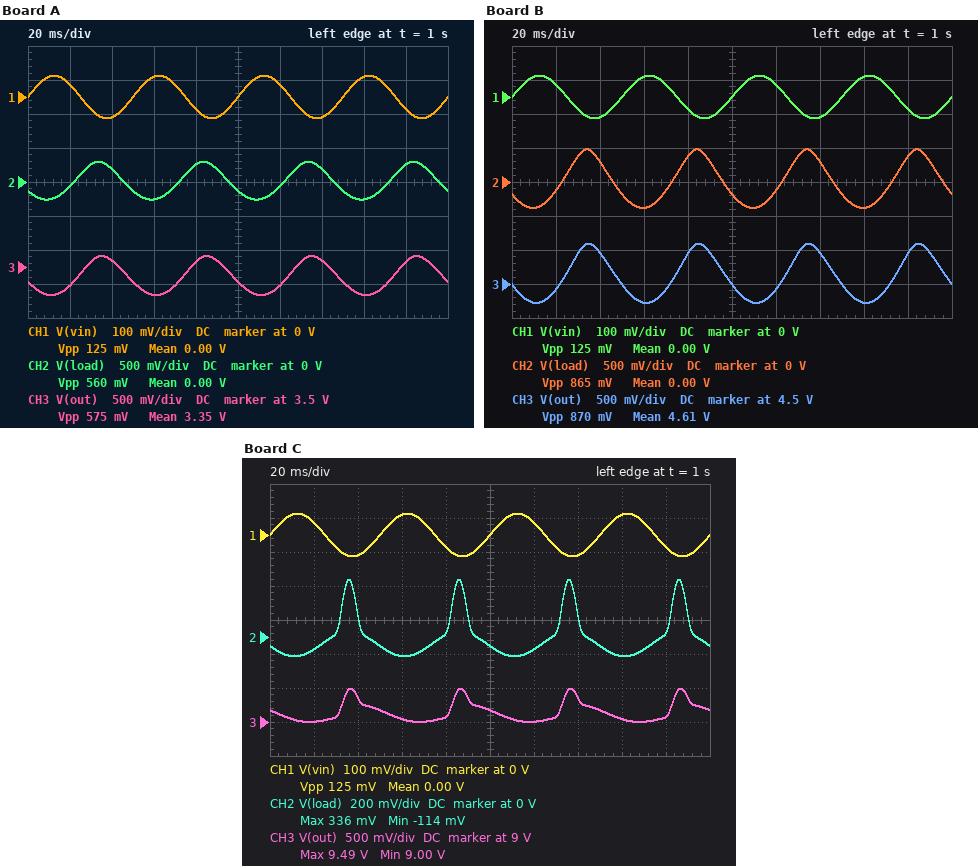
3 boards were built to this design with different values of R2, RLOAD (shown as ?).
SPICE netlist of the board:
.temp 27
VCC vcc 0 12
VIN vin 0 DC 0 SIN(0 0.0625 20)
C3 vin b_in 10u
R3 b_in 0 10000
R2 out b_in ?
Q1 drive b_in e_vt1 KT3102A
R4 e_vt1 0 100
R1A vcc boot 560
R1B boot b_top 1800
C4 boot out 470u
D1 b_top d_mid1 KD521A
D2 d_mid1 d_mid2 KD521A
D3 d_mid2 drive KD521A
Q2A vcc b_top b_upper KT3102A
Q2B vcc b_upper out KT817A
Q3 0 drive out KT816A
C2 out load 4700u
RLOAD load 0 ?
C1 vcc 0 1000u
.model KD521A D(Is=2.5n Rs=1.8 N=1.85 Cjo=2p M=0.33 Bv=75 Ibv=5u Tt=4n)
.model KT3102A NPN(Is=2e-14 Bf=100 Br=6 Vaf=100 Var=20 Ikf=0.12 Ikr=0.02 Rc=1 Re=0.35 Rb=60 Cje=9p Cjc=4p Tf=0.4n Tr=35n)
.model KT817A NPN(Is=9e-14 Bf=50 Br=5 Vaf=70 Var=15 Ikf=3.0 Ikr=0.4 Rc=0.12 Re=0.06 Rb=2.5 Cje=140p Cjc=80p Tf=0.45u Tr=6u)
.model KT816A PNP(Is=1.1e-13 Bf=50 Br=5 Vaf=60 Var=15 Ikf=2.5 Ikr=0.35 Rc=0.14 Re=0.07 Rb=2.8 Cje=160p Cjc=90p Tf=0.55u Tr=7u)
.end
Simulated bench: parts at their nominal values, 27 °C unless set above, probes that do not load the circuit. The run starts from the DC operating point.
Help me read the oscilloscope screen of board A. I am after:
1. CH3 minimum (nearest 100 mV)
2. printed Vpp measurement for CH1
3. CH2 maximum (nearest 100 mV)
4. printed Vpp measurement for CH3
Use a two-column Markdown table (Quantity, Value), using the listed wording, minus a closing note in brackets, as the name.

| Quantity | Value |
|---|---|
| CH3 minimum | 3.1 V |
| printed Vpp measurement for CH1 | 125 mV |
| CH2 maximum | 300 mV |
| printed Vpp measurement for CH3 | 575 mV |
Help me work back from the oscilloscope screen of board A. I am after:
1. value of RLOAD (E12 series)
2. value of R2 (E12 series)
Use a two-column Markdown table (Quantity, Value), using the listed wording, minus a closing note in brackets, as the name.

| Quantity | Value |
|---|---|
| value of RLOAD | 6.8 Ω |
| value of R2 | 15 kΩ |
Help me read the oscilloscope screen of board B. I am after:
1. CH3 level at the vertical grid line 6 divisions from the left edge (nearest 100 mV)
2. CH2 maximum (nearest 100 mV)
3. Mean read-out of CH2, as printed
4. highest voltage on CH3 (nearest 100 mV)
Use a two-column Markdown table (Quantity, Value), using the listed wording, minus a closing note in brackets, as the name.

| Quantity | Value |
|---|---|
| CH3 level at the vertical grid line 6 divisions from the left edge | 4.4 V |
| CH2 maximum | 500 mV |
| Mean read-out of CH2, as printed | 0.00 V |
| highest voltage on CH3 | 5.1 V |
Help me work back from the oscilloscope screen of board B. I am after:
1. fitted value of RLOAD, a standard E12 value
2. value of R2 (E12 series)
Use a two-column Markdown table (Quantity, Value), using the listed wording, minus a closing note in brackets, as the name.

| Quantity | Value |
|---|---|
| fitted value of RLOAD, a standard E12 value | 10 Ω |
| value of R2 | 27 kΩ |
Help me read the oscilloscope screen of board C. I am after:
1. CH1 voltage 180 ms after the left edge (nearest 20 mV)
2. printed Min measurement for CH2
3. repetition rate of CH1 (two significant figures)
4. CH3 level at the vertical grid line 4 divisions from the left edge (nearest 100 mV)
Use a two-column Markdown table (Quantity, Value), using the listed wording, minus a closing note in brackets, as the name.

| Quantity | Value |
|---|---|
| CH1 voltage 180 ms after the left edge | -40 mV |
| printed Min measurement for CH2 | -114 mV |
| repetition rate of CH1 | 20 Hz |
| CH3 level at the vertical grid line 4 divisions from the left edge | 9.1 V |
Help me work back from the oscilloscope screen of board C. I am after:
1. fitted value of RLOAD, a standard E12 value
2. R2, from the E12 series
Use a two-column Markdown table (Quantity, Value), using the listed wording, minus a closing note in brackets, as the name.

| Quantity | Value |
|---|---|
| fitted value of RLOAD, a standard E12 value | 2.7 Ω |
| R2, from the E12 series | 100 kΩ |
